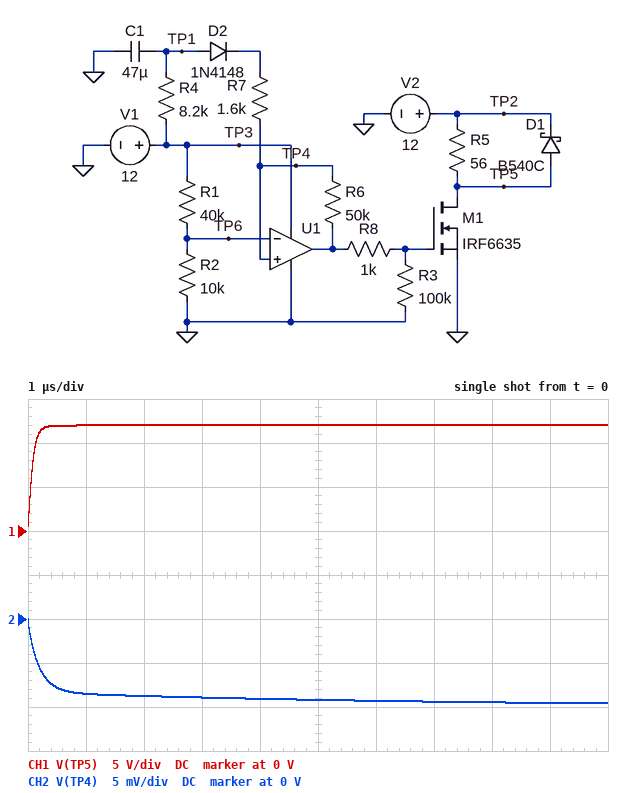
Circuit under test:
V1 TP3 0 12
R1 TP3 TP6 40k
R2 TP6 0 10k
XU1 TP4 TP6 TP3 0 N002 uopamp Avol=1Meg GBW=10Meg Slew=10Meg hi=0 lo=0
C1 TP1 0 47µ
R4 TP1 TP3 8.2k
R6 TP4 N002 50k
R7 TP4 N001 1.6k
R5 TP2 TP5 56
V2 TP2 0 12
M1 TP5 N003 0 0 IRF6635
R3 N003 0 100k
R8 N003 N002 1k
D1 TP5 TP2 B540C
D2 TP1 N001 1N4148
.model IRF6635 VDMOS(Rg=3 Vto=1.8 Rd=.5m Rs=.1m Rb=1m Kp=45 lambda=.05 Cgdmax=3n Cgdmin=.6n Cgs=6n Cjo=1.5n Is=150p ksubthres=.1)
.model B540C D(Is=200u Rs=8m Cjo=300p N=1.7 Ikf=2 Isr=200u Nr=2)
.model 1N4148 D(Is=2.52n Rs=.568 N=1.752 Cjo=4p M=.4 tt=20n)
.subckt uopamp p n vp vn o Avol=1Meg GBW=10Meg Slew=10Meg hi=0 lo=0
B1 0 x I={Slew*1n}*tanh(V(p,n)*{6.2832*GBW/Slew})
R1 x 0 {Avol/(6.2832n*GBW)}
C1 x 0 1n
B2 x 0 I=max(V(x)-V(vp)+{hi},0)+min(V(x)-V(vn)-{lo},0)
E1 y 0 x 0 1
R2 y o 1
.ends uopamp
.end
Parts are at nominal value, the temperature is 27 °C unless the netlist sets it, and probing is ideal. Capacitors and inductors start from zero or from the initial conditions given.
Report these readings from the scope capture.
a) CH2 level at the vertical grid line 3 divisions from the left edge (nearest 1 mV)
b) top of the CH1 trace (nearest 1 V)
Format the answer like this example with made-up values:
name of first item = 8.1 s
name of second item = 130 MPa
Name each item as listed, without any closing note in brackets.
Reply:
CH2 level at the vertical grid line 3 divisions from the left edge = -9 mV
top of the CH1 trace = 12 V
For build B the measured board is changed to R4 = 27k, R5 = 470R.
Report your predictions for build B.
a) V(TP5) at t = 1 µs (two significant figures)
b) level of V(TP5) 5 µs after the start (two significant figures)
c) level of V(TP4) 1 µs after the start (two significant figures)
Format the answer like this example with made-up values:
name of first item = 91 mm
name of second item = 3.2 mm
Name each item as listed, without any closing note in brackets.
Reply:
V(TP5) at t = 1 µs = 9.5 V
level of V(TP5) 5 µs after the start = 12 V
level of V(TP4) 1 µs after the start = -8.8 mV
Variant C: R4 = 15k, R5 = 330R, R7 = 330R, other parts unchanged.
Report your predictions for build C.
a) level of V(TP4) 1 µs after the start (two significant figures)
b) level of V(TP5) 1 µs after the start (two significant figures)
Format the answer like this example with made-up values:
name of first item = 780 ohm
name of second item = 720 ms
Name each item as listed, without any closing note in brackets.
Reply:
level of V(TP4) 1 µs after the start = -8.7 mV
level of V(TP5) 1 µs after the start = 11 V
